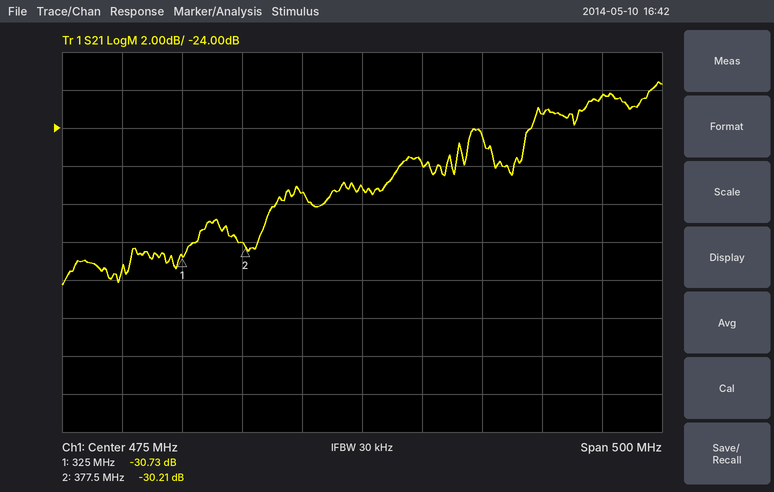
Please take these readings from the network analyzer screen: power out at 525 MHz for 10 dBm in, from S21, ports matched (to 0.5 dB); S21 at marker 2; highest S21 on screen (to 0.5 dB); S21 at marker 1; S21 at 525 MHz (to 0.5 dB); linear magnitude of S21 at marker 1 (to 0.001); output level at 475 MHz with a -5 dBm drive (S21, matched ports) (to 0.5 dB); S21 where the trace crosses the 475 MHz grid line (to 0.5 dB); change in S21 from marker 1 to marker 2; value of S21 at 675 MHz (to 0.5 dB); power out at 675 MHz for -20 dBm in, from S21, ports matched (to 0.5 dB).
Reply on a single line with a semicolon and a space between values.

-16.0 dBm; -30.21 dB; -21.5 dB; -30.73 dB; -26.0 dB; 0.029; -32.0 dBm; -27.0 dB; 0.52 dB; -22.5 dB; -42.5 dBm
